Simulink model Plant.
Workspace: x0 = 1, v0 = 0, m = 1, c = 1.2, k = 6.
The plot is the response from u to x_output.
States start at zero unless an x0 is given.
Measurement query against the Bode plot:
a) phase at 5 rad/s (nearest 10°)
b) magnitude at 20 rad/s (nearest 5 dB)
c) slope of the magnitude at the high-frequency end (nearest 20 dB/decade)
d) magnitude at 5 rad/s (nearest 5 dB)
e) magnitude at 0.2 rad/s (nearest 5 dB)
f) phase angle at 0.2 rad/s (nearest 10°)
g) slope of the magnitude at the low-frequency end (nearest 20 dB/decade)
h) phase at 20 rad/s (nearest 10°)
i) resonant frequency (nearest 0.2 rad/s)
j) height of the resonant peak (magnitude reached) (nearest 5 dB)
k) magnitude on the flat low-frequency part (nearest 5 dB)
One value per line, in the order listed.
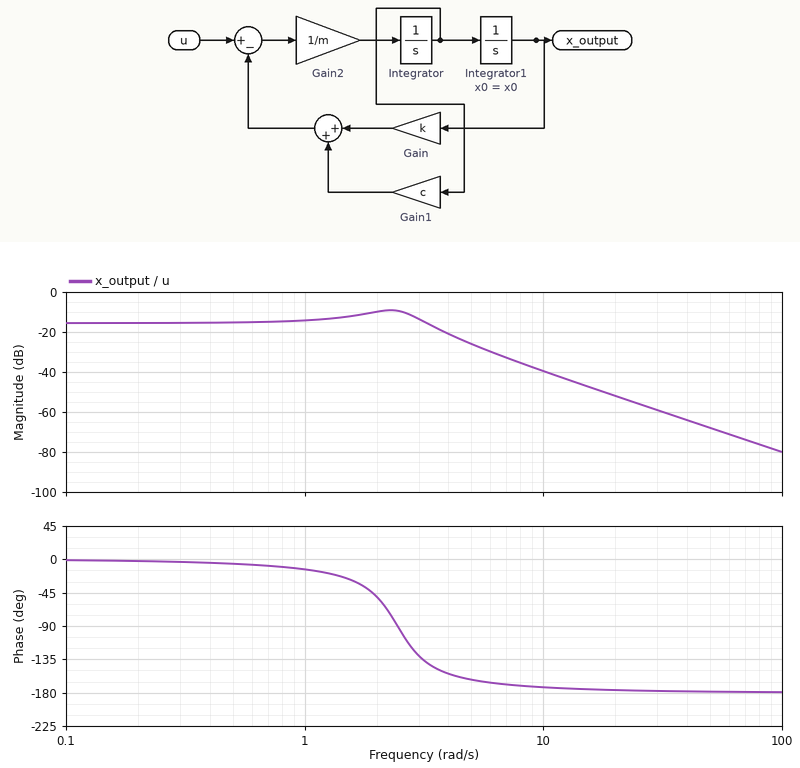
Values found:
-160°
-50 dB
-40 dB/decade
-25 dB
-15 dB
0°
0 dB/decade
-180°
2.2 rad/s
-10 dB
-15 dB
